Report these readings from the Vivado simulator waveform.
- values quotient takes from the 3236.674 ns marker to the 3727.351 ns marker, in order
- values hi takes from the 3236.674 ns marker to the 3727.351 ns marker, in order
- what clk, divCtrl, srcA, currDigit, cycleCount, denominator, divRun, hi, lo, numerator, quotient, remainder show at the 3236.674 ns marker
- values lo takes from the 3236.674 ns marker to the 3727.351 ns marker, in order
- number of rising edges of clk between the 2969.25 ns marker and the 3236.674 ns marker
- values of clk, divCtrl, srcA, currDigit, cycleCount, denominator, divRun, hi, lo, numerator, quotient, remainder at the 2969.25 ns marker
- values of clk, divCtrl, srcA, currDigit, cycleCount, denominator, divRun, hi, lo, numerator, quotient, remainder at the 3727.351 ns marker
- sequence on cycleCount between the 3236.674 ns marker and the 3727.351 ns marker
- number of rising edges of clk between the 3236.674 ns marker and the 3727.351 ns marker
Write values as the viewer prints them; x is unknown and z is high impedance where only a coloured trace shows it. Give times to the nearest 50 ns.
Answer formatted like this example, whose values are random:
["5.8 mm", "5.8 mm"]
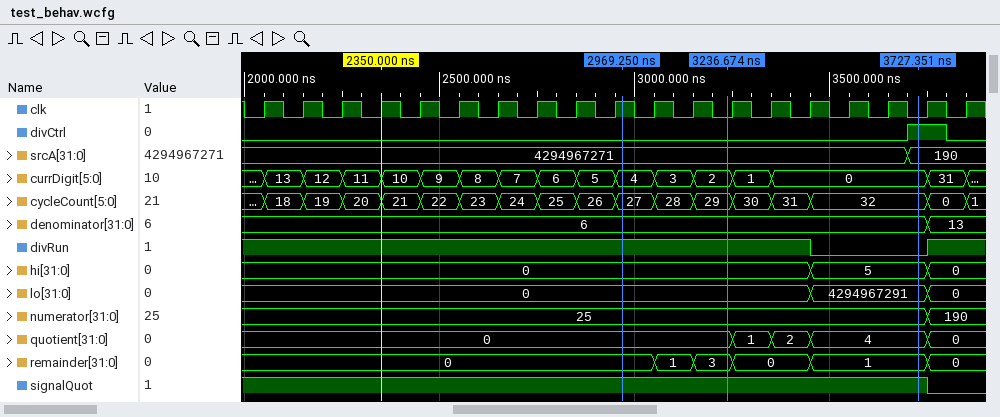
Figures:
["0, 1, 2, 4", "0, 5", "clk=0, divCtrl=0, srcA=4294967271, currDigit=2, cycleCount=29, denominator=6, divRun=1, hi=0, lo=0, numerator=25, quotient=0, remainder=3", "0, 4294967291", "2", "clk=1, divCtrl=0, srcA=4294967271, currDigit=4, cycleCount=27, denominator=6, divRun=1, hi=0, lo=0, numerator=25, quotient=0, remainder=0", "clk=0, divCtrl=1, srcA=190, currDigit=0, cycleCount=32, denominator=6, divRun=0, hi=5, lo=4294967291, numerator=25, quotient=4, remainder=1", "29, 30, 31, 32", "5"]
